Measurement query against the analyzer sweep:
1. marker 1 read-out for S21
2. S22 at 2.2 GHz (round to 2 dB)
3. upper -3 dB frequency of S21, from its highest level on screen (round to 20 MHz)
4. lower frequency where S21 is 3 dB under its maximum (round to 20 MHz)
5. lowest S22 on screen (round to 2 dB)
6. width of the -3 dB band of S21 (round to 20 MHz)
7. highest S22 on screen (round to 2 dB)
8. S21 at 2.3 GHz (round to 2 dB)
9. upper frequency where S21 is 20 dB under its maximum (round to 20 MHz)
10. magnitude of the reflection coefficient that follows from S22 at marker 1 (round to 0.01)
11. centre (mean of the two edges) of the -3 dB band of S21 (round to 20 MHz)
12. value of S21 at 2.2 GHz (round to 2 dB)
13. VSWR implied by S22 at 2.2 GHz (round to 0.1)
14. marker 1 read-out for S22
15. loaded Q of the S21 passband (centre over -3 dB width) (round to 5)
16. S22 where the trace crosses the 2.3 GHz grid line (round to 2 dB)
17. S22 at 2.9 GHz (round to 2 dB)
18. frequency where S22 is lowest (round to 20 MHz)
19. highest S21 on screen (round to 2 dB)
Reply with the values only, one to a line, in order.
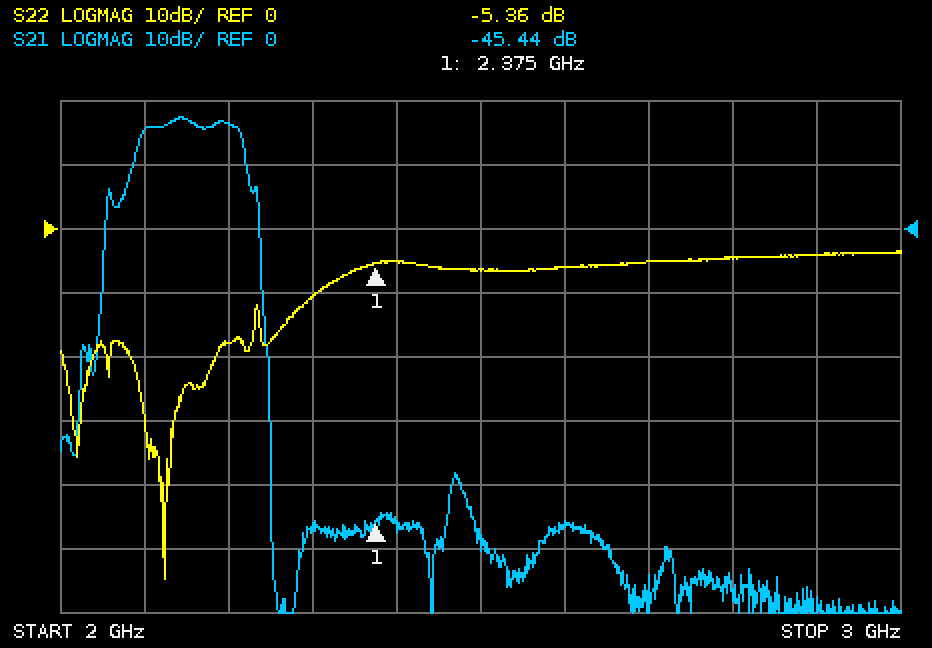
-45.44 dB
-18 dB
2.22 GHz
2.10 GHz
-54 dB
120 MHz
-4 dB
-46 dB
2.24 GHz
0.54
2.16 GHz
16 dB
1.3
-5.36 dB
20
-10 dB
-4 dB
2.12 GHz
18 dB
